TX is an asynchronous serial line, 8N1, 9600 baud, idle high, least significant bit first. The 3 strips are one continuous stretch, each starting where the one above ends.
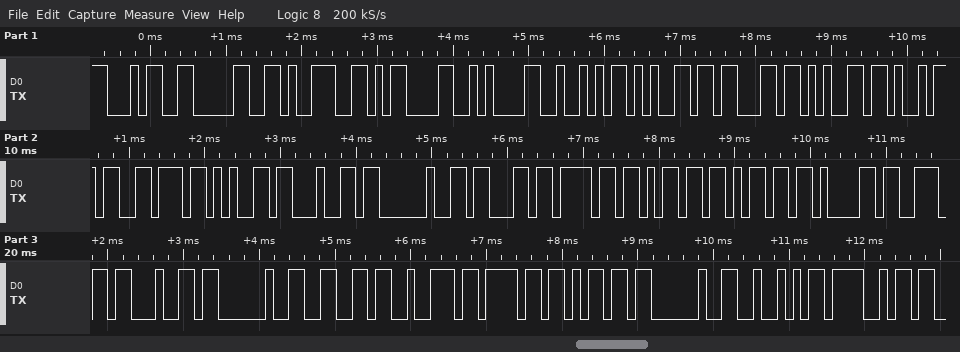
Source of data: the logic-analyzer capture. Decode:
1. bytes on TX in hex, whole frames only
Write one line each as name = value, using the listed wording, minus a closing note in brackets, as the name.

bytes on TX in hex, whole frames only = 34 30 39 0D 0A 52 65 63 65 69 76 65 64 20 63 6F 6D 6D 61 6E 64 20 66 72 6F 6D 20 52 4F
